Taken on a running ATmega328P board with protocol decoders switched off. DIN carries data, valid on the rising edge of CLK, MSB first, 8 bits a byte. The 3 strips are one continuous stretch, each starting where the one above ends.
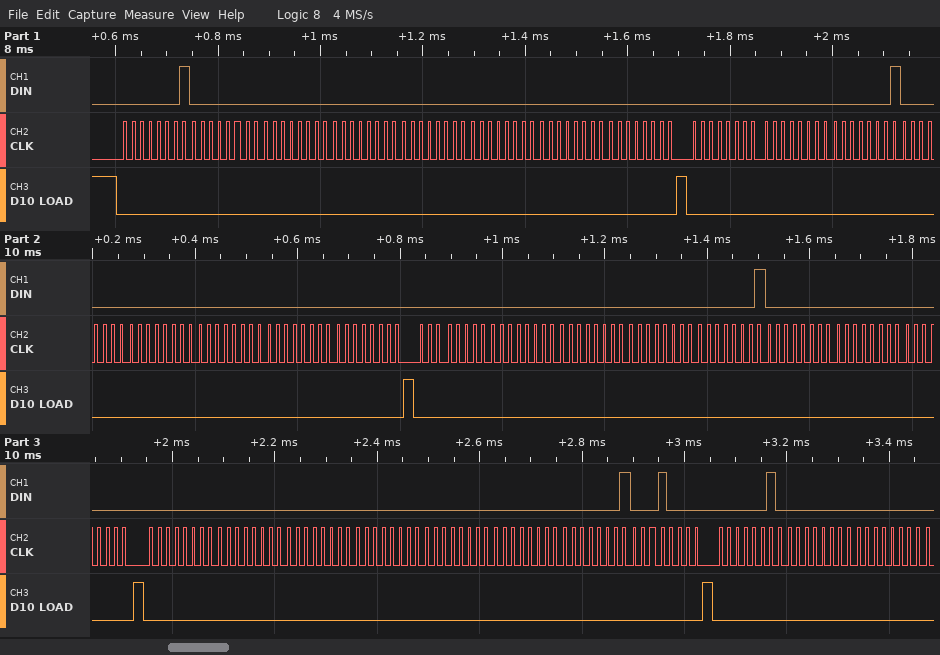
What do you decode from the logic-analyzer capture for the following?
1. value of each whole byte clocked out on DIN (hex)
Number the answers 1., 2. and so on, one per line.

1. 0x01 0x00 0x00 0x00 0x00 0x00 0x00 0x00 0x00 0x00 0x01 0x00 0x00 0x00 0x00 0x00 0x00 0x00 0x00 0x00 0x01 0x00 0x00 0x00 0x00 0x00 0x00 0x00 0x00 0x00 0x01 0x10 0x02 0x00 0x00
